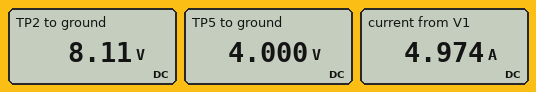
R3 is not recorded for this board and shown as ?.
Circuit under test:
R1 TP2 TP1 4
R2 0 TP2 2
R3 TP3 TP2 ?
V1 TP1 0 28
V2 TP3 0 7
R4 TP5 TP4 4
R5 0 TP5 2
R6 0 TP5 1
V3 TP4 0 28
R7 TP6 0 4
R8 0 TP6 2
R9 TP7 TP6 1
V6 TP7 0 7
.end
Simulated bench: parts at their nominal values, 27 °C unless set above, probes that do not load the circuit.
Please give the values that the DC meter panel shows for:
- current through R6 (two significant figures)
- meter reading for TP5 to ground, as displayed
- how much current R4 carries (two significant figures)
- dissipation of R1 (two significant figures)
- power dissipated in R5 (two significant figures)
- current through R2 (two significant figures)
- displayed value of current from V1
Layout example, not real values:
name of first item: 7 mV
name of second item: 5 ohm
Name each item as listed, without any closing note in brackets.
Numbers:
current through R6: 4.0 A
meter reading for TP5 to ground, as displayed: 4.000 V
how much current R4 carries: 6.0 A
dissipation of R1: 99 W
power dissipated in R5: 8.0 W
current through R2: 4.1 A
displayed value of current from V1: 4.974 A
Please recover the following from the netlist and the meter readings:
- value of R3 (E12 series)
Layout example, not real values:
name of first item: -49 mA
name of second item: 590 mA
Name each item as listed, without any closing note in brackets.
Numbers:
value of R3: 1.2 Ω
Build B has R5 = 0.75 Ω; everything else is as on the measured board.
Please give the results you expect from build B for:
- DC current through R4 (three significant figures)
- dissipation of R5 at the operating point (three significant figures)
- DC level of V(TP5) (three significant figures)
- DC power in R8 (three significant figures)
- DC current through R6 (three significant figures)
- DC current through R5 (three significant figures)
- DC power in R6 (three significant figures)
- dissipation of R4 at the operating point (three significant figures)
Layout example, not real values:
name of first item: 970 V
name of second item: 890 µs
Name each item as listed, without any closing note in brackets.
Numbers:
DC current through R4: 6.32 A
dissipation of R5 at the operating point: 9.79 W
DC level of V(TP5): 2.71 V
DC power in R8: 8.00 W
DC current through R6: 2.71 A
DC current through R5: 3.61 A
DC power in R6: 7.34 W
dissipation of R4 at the operating point: 160 W
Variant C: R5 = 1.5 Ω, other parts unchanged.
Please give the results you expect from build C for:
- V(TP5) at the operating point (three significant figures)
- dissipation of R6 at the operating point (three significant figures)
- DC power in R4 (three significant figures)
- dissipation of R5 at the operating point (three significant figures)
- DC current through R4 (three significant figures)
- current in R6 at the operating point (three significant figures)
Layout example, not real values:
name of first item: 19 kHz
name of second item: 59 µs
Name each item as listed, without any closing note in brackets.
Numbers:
V(TP5) at the operating point: 3.65 V
dissipation of R6 at the operating point: 13.3 W
DC power in R4: 148 W
dissipation of R5 at the operating point: 8.89 W
DC current through R4: 6.09 A
current in R6 at the operating point: 3.65 A
